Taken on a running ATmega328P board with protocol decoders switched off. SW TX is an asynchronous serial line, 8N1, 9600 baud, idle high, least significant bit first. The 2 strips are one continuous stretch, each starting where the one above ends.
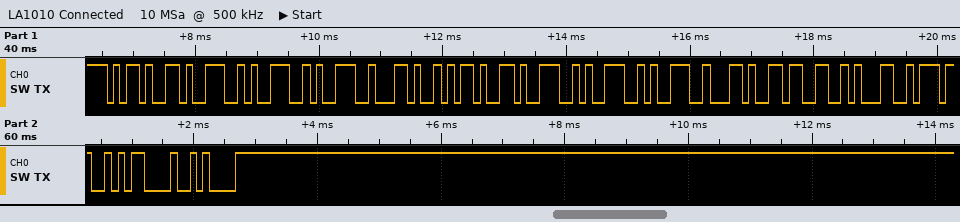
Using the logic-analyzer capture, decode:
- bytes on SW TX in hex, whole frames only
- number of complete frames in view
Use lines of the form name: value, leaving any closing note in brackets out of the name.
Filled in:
bytes on SW TX in hex, whole frames only: 0x2D 0x39 0x39 0x39 0x2C 0x2D 0x39 0x39 0x39 0x2C 0x33 0x31 0x37 0x0D 0x0A
number of complete frames in view: 15
